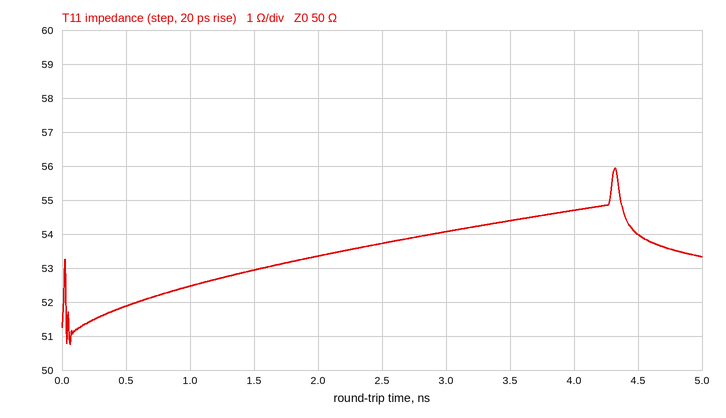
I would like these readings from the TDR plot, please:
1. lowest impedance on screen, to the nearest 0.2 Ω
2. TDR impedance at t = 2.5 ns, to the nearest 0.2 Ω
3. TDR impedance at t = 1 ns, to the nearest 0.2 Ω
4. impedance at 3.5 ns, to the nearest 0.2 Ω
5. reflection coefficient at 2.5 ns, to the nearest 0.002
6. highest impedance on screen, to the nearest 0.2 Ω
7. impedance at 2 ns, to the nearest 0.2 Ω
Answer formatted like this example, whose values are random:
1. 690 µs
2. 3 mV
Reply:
1. 50.8 Ω
2. 53.8 Ω
3. 52.4 Ω
4. 54.4 Ω
5. +0.036
6. 56.0 Ω
7. 53.4 Ω
